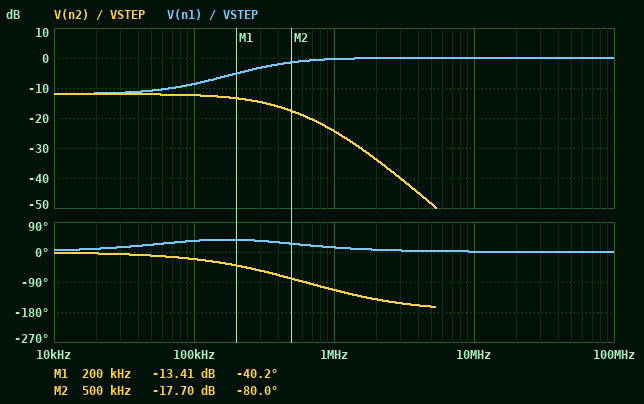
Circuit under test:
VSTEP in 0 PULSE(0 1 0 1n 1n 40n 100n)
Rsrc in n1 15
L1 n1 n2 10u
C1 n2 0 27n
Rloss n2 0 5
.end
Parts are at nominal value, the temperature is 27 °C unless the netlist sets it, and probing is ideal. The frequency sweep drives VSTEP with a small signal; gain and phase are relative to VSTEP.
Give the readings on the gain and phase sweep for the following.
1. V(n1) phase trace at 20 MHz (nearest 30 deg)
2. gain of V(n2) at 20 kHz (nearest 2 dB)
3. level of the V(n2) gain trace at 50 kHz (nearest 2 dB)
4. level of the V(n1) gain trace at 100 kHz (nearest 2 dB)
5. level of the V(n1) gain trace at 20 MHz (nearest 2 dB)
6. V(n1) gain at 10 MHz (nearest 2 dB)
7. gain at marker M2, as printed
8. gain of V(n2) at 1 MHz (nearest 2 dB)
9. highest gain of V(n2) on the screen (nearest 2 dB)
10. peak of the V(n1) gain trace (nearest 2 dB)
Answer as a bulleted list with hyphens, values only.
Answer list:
- 0 deg
- -12 dB
- -12 dB
- -8 dB
- 0 dB
- 0 dB
- -17.70 dB
- -24 dB
- -12 dB
- 0 dB
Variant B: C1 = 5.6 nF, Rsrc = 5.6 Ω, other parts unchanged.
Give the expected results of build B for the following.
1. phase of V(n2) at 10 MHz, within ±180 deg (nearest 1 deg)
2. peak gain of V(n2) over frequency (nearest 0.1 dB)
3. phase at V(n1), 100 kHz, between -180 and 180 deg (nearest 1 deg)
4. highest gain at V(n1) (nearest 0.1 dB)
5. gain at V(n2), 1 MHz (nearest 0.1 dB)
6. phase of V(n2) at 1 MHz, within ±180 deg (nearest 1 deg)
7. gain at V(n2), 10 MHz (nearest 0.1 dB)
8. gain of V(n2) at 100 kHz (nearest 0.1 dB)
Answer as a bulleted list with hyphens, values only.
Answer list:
- -150 deg
- -6.5 dB
- 21 deg
- 0 dB
- -22.1 dB
- -90 deg
- -48.1 dB
- -7.8 dB
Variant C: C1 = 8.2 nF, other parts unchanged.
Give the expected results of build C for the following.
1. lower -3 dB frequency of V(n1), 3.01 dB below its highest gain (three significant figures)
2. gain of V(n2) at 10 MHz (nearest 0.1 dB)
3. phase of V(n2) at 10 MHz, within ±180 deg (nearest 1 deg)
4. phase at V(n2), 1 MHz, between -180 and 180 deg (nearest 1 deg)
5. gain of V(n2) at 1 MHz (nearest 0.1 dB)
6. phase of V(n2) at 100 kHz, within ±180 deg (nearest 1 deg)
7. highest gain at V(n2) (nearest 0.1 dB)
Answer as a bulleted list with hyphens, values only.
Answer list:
- 304 kHz
- -50.8 dB
- -157 deg
- -87 deg
- -22.5 dB
- -19 deg
- -12.0 dB
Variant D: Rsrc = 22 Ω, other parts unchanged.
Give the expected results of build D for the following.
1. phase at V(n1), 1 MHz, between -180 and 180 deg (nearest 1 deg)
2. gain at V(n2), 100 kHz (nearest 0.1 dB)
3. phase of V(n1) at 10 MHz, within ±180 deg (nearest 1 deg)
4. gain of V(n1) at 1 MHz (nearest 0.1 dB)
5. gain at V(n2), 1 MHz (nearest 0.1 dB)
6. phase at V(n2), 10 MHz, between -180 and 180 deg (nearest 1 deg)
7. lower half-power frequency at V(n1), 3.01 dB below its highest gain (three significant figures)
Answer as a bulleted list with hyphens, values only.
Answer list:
- 20 deg
- -14.9 dB
- 2 deg
- -0.7 dB
- -24.7 dB
- -171 deg
- 434 kHz
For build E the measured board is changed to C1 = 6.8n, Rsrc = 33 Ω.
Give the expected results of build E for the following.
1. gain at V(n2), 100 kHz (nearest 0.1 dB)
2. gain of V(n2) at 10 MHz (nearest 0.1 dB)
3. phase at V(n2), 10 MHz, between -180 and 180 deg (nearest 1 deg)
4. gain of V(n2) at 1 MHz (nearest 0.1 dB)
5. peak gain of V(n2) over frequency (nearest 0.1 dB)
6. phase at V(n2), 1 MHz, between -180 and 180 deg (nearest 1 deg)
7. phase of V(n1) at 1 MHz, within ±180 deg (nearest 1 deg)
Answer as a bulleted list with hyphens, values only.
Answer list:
- -17.7 dB
- -49.4 dB
- -152 deg
- -23.4 dB
- -17.6 dB
- -71 deg
- 27 deg
